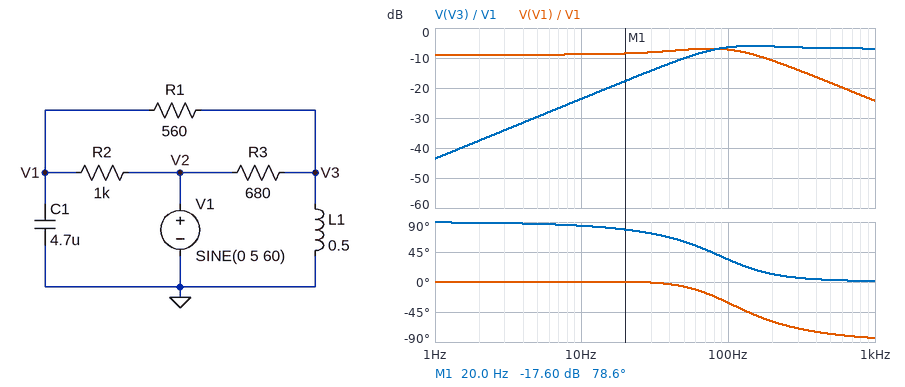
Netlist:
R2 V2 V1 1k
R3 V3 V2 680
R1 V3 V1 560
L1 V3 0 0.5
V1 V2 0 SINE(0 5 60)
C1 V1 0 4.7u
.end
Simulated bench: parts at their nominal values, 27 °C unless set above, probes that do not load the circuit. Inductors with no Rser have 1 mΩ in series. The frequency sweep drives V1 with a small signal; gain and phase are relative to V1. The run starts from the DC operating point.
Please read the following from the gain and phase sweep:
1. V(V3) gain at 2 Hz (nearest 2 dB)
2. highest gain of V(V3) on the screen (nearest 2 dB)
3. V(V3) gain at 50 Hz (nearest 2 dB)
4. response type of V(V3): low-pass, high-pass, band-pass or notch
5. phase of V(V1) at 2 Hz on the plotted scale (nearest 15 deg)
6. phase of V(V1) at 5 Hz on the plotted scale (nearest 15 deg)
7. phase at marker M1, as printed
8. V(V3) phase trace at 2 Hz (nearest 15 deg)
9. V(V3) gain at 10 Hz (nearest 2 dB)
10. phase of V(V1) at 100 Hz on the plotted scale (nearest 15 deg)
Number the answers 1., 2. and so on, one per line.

1. -38 dB
2. -6 dB
3. -10 dB
4. high-pass
5. 0 deg
6. 0 deg
7. 78.6 deg
8. 90 deg
9. -24 dB
10. -30 deg
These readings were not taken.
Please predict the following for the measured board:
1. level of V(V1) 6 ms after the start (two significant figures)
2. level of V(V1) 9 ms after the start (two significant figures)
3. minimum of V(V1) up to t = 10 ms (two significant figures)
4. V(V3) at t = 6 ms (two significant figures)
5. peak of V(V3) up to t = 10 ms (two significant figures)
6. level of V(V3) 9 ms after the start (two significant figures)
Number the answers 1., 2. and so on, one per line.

1. 1.9 V
2. -120 mV
3. -930 mV
4. -130 mV
5. 1.3 V
6. -1.7 V
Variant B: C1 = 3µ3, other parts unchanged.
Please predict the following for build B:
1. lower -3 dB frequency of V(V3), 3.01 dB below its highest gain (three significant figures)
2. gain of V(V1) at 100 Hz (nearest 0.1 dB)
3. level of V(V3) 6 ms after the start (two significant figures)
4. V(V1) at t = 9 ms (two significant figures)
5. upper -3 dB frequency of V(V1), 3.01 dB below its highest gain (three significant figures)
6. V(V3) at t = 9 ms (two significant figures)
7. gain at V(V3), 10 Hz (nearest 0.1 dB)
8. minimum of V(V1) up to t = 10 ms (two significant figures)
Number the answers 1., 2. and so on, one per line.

1. 65.1 Hz
2. -5.5 dB
3. -220 mV
4. -540 mV
5. 215 Hz
6. -1.8 V
7. -23.6 dB
8. -1.4 V
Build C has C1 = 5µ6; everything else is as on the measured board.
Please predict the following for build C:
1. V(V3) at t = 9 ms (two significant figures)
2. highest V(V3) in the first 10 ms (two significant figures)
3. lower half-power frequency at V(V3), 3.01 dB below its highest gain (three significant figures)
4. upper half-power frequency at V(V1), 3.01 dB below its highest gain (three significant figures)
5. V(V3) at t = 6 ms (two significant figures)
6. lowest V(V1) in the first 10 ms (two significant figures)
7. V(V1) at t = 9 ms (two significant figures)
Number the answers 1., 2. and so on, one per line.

1. -1.6 V
2. 1.2 V
3. 56.1 Hz
4. 155 Hz
5. -96 mV
6. -690 mV
7. 84 mV
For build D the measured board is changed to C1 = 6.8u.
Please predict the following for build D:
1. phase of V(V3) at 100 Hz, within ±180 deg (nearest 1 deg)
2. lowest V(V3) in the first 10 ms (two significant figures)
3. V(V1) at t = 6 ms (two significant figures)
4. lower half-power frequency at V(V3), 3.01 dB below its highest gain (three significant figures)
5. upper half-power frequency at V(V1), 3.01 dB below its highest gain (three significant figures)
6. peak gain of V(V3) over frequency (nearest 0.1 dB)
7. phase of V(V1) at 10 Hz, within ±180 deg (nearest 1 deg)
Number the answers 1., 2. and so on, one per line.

1. 32 deg
2. -1.7 V
3. 1.8 V
4. 55.3 Hz
5. 135 Hz
6. -6.8 dB
7. -2 deg
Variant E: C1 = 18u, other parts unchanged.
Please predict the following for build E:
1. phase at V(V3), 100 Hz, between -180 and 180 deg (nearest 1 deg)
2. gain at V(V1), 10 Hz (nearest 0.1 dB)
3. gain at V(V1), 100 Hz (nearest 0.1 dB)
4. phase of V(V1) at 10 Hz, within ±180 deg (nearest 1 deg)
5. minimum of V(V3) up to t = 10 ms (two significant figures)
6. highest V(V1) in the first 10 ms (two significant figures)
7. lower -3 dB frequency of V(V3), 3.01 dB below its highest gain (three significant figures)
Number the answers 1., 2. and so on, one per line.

1. 37 deg
2. -9.3 dB
3. -17.5 dB
4. -16 deg
5. -1.4 V
6. 1.1 V
7. 80.7 Hz
